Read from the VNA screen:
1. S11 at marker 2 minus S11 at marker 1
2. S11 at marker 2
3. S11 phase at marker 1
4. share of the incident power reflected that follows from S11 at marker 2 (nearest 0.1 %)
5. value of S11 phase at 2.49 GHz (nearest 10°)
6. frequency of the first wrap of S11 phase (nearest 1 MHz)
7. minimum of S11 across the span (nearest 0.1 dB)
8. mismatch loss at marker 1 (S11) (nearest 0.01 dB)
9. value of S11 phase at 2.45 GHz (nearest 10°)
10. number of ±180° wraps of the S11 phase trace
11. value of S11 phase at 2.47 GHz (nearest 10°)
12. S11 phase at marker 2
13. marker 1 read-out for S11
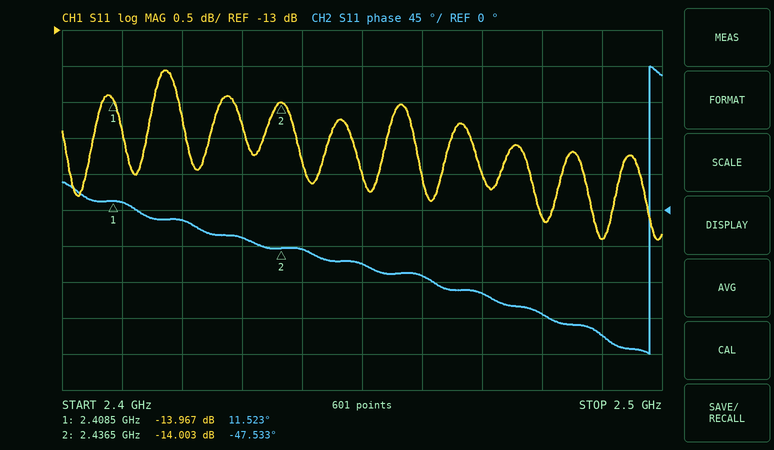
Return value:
-0.036 dB
-14.003 dB
11.523°
4.0 %
-160°
2.498 GHz
-15.9 dB
0.18 dB
-70°
1
-100°
-47.533°
-13.967 dB
